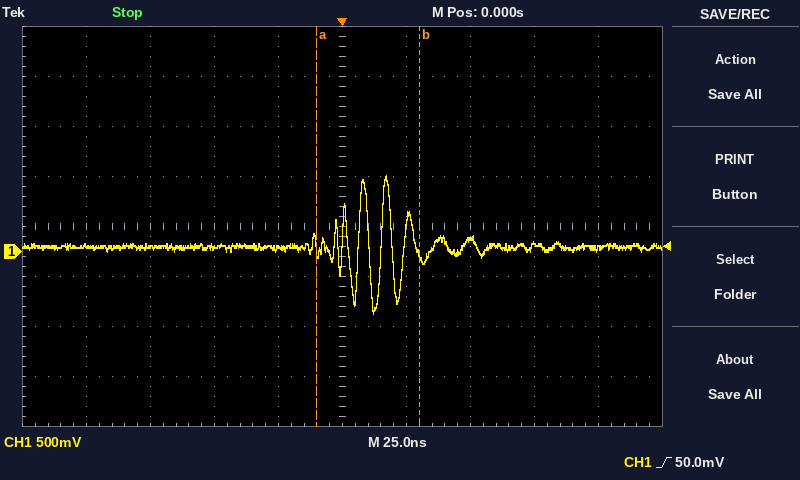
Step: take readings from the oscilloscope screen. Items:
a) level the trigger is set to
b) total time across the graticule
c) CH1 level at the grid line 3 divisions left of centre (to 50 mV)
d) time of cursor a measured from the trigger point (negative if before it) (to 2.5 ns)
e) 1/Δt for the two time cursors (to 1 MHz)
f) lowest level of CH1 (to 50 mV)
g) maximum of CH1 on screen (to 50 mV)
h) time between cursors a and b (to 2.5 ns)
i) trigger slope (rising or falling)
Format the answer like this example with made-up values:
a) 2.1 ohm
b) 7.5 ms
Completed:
a) 50.0 mV
b) 250 ns
c) 50 mV
d) -10.0 ns
e) 25 MHz
f) -600 mV
g) 750 mV
h) 40.0 ns
i) rising
